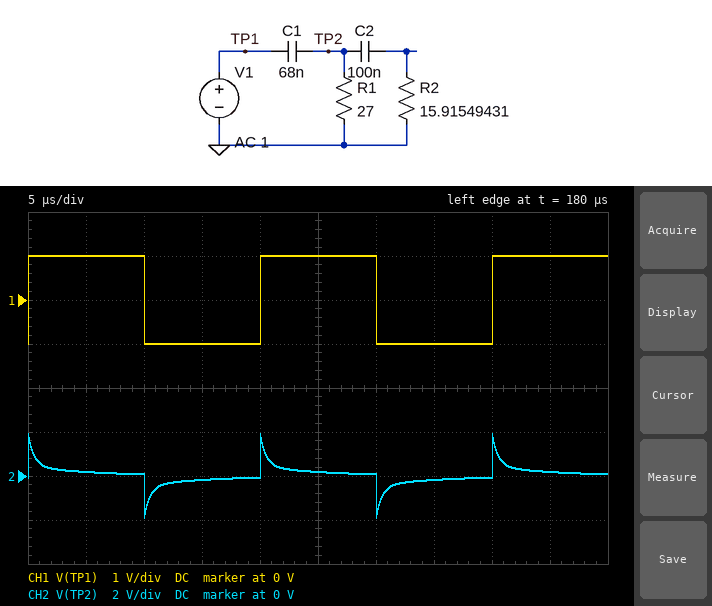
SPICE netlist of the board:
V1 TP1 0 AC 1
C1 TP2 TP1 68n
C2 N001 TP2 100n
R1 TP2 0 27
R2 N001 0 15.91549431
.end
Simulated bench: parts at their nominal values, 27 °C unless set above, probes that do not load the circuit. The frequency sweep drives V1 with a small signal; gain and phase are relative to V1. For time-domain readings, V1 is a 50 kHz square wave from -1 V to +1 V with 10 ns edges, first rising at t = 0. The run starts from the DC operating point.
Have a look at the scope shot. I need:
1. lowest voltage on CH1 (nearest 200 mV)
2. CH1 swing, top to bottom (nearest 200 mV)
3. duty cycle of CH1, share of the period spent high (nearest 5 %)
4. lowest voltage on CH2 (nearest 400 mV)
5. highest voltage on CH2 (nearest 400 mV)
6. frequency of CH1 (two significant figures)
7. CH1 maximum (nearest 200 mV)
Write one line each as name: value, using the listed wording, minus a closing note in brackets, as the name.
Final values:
lowest voltage on CH1: -1.0 V
CH1 swing, top to bottom: 2.0 V
duty cycle of CH1, share of the period spent high: 50 %
lowest voltage on CH2: -2.0 V
highest voltage on CH2: 2.0 V
frequency of CH1: 50 kHz
CH1 maximum: 1.0 V
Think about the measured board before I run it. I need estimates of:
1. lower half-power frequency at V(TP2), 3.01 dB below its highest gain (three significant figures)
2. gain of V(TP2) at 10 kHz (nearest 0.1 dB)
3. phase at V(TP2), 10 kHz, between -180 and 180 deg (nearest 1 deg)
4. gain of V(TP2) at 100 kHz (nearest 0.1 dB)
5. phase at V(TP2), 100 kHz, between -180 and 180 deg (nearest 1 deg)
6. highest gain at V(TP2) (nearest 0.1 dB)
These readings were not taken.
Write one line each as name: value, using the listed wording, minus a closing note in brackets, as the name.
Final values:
lower half-power frequency at V(TP2), 3.01 dB below its highest gain: 274 kHz
gain of V(TP2) at 10 kHz: -19.2 dB
phase at V(TP2), 10 kHz, between -180 and 180 deg: 74 deg
gain of V(TP2) at 100 kHz: -7.5 dB
phase at V(TP2), 100 kHz, between -180 and 180 deg: 43 deg
highest gain at V(TP2): 0 dB
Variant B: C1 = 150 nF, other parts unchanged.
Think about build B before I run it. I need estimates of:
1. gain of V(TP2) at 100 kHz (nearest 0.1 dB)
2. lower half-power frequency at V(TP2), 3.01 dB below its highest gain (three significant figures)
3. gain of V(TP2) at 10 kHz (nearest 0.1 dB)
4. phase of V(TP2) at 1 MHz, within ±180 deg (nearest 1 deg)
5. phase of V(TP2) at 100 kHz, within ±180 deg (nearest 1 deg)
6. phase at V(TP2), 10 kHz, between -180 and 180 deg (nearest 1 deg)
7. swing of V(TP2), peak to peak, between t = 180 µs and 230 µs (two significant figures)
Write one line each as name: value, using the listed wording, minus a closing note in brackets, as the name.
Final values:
gain of V(TP2) at 100 kHz: -3.6 dB
lower half-power frequency at V(TP2), 3.01 dB below its highest gain: 125 kHz
gain of V(TP2) at 10 kHz: -12.7 dB
phase of V(TP2) at 1 MHz, within ±180 deg: 6 deg
phase of V(TP2) at 100 kHz, within ±180 deg: 29 deg
phase at V(TP2), 10 kHz, between -180 and 180 deg: 67 deg
swing of V(TP2), peak to peak, between t = 180 µs and 230 µs: 3.6 V
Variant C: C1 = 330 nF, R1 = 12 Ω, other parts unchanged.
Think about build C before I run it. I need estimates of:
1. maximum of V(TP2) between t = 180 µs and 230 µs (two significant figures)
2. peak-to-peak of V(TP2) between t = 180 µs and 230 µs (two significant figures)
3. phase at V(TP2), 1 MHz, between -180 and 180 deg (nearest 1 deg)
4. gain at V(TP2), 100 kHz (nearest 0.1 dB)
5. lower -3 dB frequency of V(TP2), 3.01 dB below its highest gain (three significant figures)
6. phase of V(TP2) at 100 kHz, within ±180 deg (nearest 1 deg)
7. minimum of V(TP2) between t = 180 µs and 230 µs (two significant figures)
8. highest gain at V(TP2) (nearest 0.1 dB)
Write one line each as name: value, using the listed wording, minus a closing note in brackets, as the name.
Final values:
maximum of V(TP2) between t = 180 µs and 230 µs: 1.8 V
peak-to-peak of V(TP2) between t = 180 µs and 230 µs: 3.6 V
phase at V(TP2), 1 MHz, between -180 and 180 deg: 4 deg
gain at V(TP2), 100 kHz: -2.1 dB
lower -3 dB frequency of V(TP2), 3.01 dB below its highest gain: 67.6 kHz
phase of V(TP2) at 100 kHz, within ±180 deg: 26 deg
minimum of V(TP2) between t = 180 µs and 230 µs: -1.8 V
highest gain at V(TP2): 0 dB
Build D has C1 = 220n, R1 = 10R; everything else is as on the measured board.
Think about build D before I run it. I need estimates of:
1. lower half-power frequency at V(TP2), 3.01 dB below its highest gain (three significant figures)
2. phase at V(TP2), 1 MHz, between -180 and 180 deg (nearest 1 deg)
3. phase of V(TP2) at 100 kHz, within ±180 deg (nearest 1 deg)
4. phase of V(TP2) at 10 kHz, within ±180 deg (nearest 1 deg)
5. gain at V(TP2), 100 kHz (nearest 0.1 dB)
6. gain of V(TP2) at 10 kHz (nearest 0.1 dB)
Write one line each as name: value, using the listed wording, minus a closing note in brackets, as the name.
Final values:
lower half-power frequency at V(TP2), 3.01 dB below its highest gain: 127 kHz
phase at V(TP2), 1 MHz, between -180 and 180 deg: 7 deg
phase of V(TP2) at 100 kHz, within ±180 deg: 38 deg
phase of V(TP2) at 10 kHz, within ±180 deg: 79 deg
gain at V(TP2), 100 kHz: -3.8 dB
gain of V(TP2) at 10 kHz: -17.4 dB
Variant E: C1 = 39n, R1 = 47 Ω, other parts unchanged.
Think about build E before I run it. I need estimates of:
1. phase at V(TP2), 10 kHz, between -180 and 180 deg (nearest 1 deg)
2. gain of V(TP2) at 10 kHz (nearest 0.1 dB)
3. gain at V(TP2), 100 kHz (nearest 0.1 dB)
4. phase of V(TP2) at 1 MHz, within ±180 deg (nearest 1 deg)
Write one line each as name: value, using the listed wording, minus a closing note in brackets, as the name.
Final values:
phase at V(TP2), 10 kHz, between -180 and 180 deg: 68 deg
gain of V(TP2) at 10 kHz: -19.7 dB
gain at V(TP2), 100 kHz: -9.9 dB
phase of V(TP2) at 1 MHz, within ±180 deg: 18 deg
